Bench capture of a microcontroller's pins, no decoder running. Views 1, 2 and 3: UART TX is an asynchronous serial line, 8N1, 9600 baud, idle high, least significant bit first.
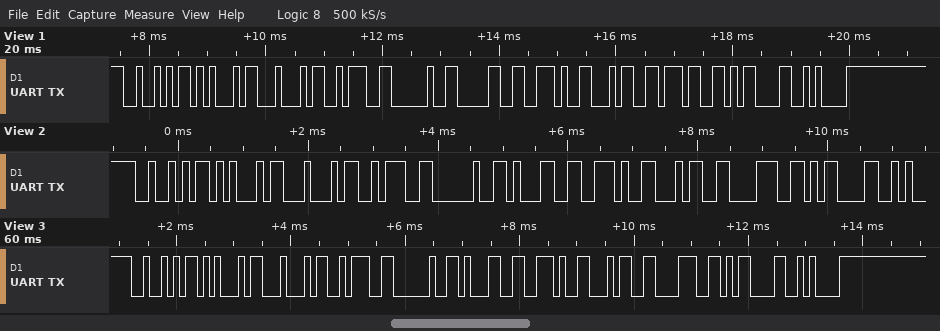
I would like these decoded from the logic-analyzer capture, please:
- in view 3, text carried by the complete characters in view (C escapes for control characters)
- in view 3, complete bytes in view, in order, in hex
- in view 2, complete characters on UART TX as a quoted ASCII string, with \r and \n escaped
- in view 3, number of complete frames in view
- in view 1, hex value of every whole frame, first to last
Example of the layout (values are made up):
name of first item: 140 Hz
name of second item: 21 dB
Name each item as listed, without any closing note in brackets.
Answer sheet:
in view 3, text carried by the complete characters in view: "RED: 1.48\r\n"
in view 3, complete bytes in view, in order, in hex: 52 45 44 3A 20 31 2E 34 38 0D 0A
in view 2, complete characters on UART TX as a quoted ASCII string, with \r and \n escaped: "RED: 1.48\r"
in view 3, number of complete frames in view: 11
in view 1, hex value of every whole frame, first to last: 52 45 44 3A 20 30 2E 34 37 0D 0A
